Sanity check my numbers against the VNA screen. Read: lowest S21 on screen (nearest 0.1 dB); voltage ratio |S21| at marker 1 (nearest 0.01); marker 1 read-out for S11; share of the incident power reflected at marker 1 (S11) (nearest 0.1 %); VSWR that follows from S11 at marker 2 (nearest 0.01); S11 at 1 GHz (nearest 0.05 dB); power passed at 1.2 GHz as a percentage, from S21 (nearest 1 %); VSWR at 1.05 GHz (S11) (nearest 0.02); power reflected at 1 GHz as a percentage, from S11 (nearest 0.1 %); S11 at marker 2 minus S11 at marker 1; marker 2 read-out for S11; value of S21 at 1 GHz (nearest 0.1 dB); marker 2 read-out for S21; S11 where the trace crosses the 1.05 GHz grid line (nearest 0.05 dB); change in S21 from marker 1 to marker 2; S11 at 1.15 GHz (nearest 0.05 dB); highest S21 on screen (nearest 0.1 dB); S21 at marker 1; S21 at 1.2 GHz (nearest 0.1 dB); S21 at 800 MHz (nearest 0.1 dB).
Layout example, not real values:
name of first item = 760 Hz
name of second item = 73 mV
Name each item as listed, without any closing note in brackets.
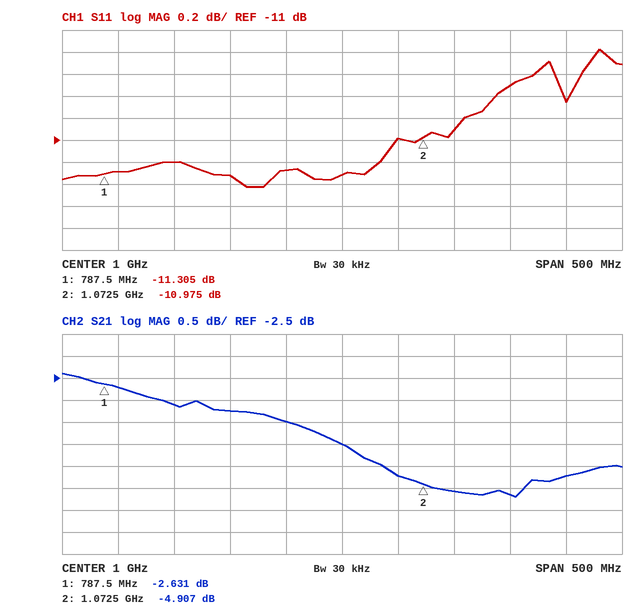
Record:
lowest S21 on screen = -5.2 dB
voltage ratio |S21| at marker 1 = 0.74
marker 1 read-out for S11 = -11.305 dB
share of the incident power reflected at marker 1 (S11) = 7.4 %
VSWR that follows from S11 at marker 2 = 1.79
S11 at 1 GHz = -11.30 dB
power passed at 1.2 GHz as a percentage, from S21 = 34 %
VSWR at 1.05 GHz (S11) = 1.78
power reflected at 1 GHz as a percentage, from S11 = 7.4 %
S11 at marker 2 minus S11 at marker 1 = 0.330 dB
marker 2 read-out for S11 = -10.975 dB
value of S21 at 1 GHz = -4.0 dB
marker 2 read-out for S21 = -4.907 dB
S11 where the trace crosses the 1.05 GHz grid line = -11.00 dB
change in S21 from marker 1 to marker 2 = -2.276 dB
S11 at 1.15 GHz = -10.50 dB
highest S21 on screen = -2.4 dB
S21 at marker 1 = -2.631 dB
S21 at 1.2 GHz = -4.7 dB
S21 at 800 MHz = -2.7 dB
